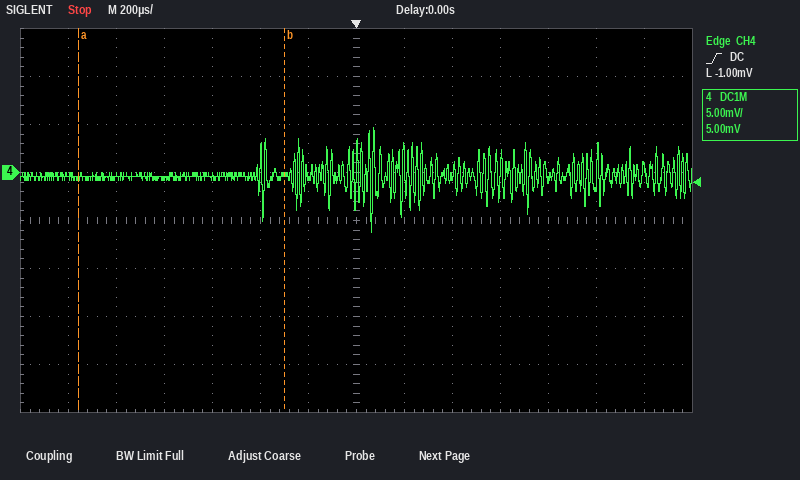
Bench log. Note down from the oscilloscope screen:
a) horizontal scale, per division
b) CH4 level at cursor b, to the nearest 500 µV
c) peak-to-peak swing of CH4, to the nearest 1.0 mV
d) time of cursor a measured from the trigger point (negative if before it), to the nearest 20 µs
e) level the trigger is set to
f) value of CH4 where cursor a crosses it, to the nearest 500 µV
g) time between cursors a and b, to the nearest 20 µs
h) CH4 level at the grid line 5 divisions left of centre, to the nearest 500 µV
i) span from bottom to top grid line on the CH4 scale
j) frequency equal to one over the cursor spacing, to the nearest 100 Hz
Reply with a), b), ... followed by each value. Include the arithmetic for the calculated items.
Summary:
a) 200 µs
b) 0.0 mV
c) 11.0 mV
d) -1.16 ms
e) -1.00 mV
f) -500 µV
g) 860 µs
h) -500 µV
i) 40 mV
j) 1 / 860 µs ≈ 1.2 kHz
